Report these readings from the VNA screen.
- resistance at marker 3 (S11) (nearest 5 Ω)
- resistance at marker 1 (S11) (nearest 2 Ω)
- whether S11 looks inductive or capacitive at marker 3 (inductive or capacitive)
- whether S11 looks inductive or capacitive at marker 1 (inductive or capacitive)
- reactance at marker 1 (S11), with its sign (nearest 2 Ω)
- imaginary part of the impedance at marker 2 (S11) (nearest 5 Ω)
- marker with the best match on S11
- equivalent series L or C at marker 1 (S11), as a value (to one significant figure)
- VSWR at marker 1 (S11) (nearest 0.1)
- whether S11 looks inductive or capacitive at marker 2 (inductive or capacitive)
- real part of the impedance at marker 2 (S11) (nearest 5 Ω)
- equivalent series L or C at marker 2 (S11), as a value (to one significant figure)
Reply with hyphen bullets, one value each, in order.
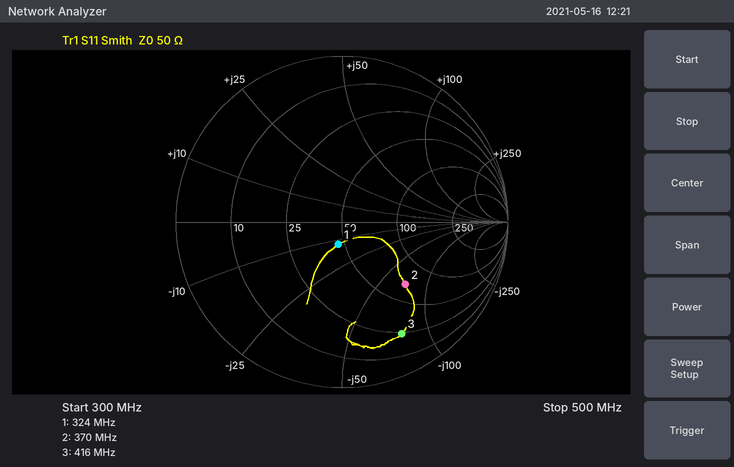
- 25 Ω
- 46 Ω
- capacitive
- capacitive
- -12 Ω
- -70 Ω
- marker 1
- 40 pF
- 1.3
- capacitive
- 70 Ω
- 6 pF
